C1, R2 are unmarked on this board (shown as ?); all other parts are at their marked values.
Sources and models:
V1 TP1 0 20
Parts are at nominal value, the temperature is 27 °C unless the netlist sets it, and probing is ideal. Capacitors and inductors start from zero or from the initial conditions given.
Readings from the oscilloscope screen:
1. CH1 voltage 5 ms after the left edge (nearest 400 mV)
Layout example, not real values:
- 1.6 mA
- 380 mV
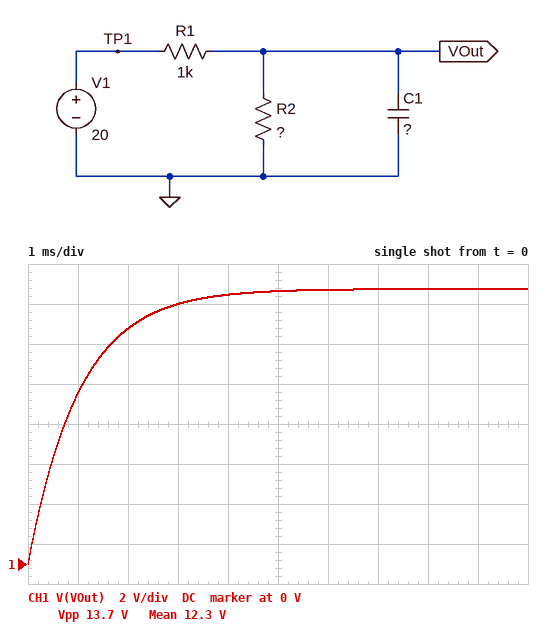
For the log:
- 13.6 V
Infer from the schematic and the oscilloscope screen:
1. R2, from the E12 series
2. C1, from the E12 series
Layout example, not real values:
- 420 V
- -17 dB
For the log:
- 2.2 kΩ
- 1.5 µF
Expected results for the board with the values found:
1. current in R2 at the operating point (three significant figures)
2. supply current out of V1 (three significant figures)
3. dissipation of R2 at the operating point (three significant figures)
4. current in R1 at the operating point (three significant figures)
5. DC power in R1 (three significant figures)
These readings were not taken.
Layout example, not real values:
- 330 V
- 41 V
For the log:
- 6.25 mA
- 6.25 mA
- 85.9 mW
- 6.25 mA
- 39.1 mW
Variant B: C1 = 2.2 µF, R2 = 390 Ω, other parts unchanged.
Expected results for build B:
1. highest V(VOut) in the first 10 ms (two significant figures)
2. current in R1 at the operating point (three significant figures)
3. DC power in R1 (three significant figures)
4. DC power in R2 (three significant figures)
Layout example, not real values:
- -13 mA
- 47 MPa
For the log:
- 5.6 V
- 14.4 mA
- 207 mW
- 80.7 mW
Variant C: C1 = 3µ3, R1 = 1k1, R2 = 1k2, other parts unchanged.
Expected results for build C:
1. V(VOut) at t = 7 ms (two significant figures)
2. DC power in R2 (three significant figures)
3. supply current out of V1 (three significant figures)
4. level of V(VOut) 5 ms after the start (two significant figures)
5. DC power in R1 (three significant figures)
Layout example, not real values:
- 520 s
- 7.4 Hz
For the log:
- 10 V
- 90.7 mW
- 8.70 mA
- 9.7 V
- 83.2 mW
